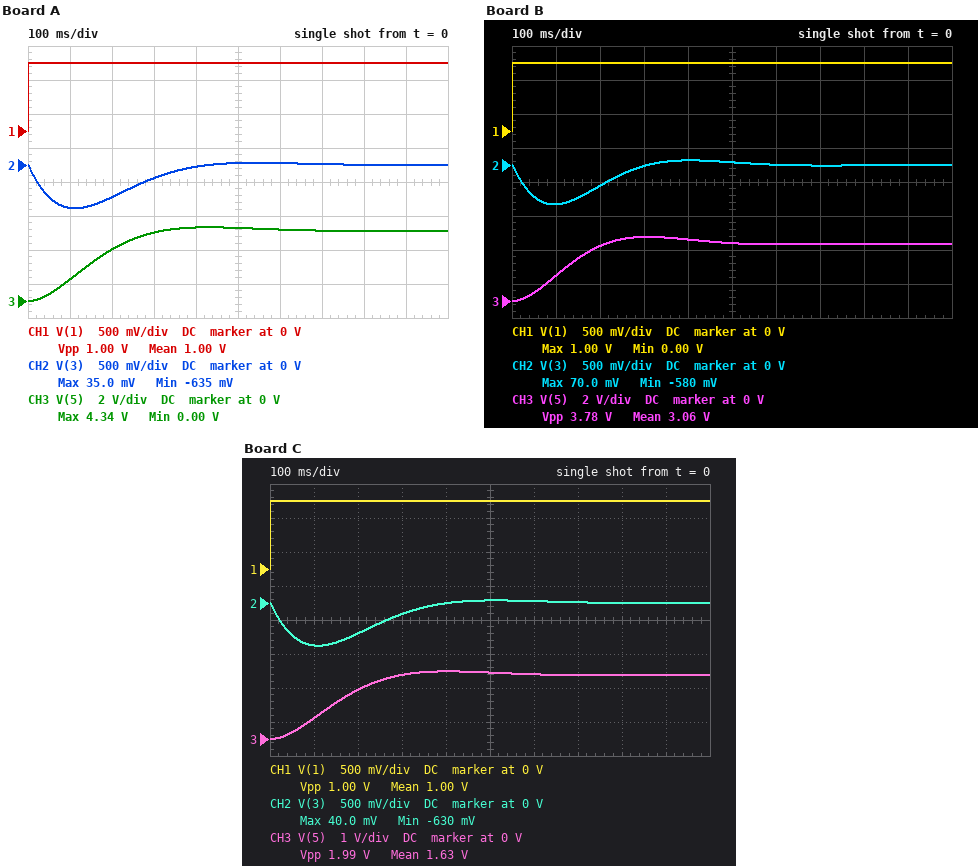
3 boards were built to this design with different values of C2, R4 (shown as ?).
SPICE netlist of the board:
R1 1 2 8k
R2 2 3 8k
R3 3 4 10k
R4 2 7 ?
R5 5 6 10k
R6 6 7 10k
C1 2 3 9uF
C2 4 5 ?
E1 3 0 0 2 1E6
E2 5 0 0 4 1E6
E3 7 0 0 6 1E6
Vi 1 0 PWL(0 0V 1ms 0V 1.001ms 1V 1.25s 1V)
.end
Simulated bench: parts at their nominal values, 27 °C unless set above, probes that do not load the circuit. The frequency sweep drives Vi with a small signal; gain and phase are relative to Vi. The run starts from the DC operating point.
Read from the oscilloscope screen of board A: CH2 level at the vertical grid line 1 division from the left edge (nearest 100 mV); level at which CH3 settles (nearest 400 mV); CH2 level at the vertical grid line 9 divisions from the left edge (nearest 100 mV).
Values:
-600 mV
4.0 V
0 V
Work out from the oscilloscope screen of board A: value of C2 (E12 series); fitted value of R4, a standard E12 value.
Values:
3.3 µF
33 kΩ
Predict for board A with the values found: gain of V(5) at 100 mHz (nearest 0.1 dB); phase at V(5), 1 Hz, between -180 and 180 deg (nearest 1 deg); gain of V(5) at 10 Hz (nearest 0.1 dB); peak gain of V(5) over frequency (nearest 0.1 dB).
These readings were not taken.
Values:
12.3 dB
-54 deg
-19.4 dB
12.3 dB
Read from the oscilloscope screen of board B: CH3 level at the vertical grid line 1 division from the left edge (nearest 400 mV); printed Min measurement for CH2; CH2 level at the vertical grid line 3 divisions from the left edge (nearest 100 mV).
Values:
1.6 V
-580 mV
0 V
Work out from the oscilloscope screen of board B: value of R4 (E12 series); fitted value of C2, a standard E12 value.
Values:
27 kΩ
2.7 µF
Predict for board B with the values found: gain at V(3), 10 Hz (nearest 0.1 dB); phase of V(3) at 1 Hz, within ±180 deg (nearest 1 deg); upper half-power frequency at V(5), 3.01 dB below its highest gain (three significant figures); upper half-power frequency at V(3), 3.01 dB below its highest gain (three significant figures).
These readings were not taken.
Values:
-13.0 dB
-128 deg
2.24 Hz
3.36 Hz
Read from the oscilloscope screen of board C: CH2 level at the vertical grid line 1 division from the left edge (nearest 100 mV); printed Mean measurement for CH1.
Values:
-600 mV
1.00 V
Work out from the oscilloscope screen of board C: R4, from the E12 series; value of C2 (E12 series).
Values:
15 kΩ
6.8 µF
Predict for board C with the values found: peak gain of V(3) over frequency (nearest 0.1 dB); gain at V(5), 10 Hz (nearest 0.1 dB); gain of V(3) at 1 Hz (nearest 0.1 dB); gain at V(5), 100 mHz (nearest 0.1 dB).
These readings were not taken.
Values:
0 dB
-25.7 dB
-2.1 dB
5.5 dB
